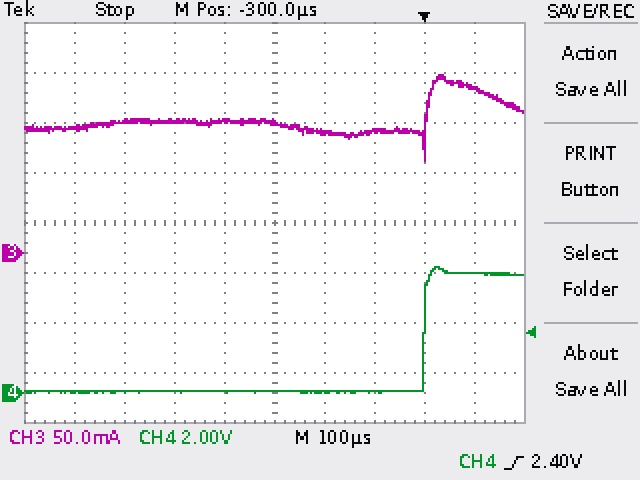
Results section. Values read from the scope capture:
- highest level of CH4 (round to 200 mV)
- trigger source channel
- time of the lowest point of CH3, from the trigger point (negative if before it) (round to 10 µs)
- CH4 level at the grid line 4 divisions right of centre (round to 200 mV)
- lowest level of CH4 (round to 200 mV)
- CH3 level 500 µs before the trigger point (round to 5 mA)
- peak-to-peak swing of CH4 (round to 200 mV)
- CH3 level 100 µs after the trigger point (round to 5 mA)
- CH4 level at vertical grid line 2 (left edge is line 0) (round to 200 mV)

5.0 V
CH4
0 µs
4.8 V
0.0 V
130 mA
5.0 V
165 mA
0.0 V
